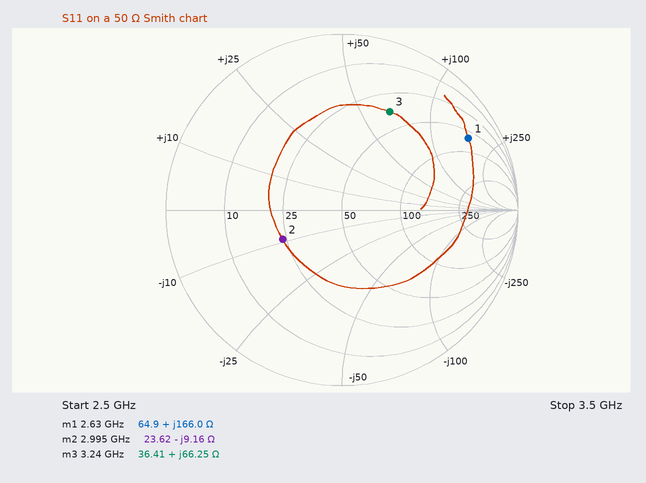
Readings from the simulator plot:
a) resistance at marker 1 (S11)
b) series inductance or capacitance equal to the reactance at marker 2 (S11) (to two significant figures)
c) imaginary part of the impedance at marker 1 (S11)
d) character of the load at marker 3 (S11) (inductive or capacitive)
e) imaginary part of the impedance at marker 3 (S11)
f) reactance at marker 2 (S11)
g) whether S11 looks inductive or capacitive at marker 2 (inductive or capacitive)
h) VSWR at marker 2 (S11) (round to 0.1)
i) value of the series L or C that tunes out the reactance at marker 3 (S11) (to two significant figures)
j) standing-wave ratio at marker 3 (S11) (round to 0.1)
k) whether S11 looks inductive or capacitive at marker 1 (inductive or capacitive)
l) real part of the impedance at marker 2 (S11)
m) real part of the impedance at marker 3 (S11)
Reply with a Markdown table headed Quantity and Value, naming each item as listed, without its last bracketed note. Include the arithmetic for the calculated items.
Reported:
| Quantity | Value |
|---|---|
| resistance at marker 1 | 64.9 Ω |
| series inductance or capacitance equal to the reactance at marker 2 (S11) | C = 1/(2π × 2.995 GHz × 9.16 Ω) ≈ 5.8 pF |
| imaginary part of the impedance at marker 1 | +166.0 Ω |
| character of the load at marker 3 (S11) | inductive |
| imaginary part of the impedance at marker 3 | +66.25 Ω |
| reactance at marker 2 | -9.16 Ω |
| whether S11 looks inductive or capacitive at marker 2 | capacitive |
| VSWR at marker 2 (S11) | 2.2 |
| value of the series L or C that tunes out the reactance at marker 3 (S11) | C = 1/(2π × 3.24 GHz × 66.25 Ω) ≈ 741 fF, so 740 fF to two significant figures |
| standing-wave ratio at marker 3 (S11) | 4.3 |
| whether S11 looks inductive or capacitive at marker 1 | inductive |
| real part of the impedance at marker 2 | 23.62 Ω |
| real part of the impedance at marker 3 | 36.41 Ω |
